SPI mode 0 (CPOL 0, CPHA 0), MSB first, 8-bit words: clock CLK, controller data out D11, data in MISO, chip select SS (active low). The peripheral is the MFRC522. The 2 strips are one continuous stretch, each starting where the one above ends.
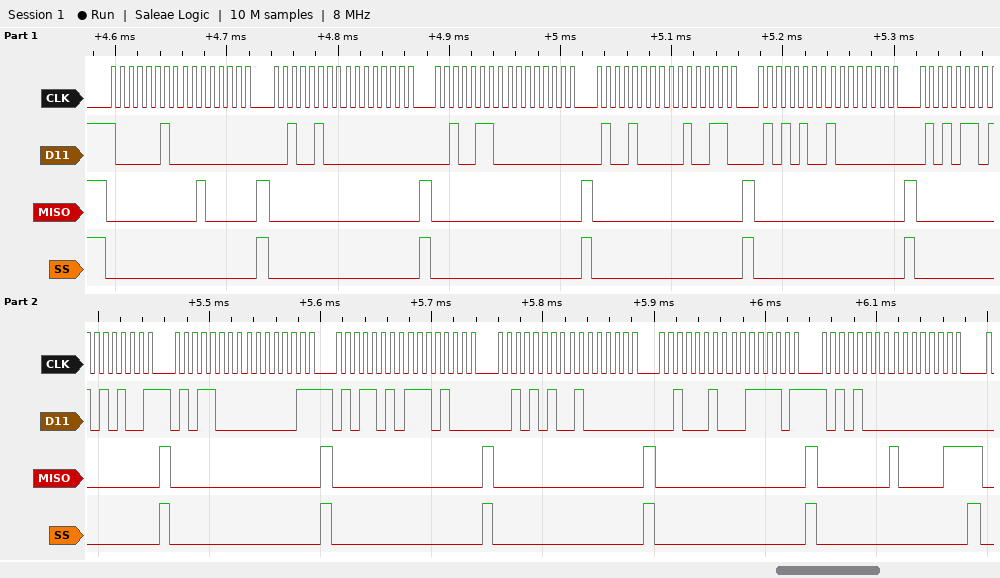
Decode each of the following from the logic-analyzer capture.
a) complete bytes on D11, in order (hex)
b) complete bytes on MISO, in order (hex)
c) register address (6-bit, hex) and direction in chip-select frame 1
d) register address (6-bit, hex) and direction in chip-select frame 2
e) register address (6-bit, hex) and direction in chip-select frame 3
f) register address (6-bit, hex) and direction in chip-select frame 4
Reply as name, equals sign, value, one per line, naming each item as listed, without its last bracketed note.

complete bytes on D11, in order = 82 00 24 00 26 00 48 26 54 80 56 A9 58 03 5A E8 2A 40 22 3D A8 00
complete bytes on MISO, in order = 00 20 00 00 00 00 00 00 00 00 00 00 00 00 00 00 00 00 00 00 00 83
register address (6-bit, hex) and direction in chip-select frame 1 = 0x01 read
register address (6-bit, hex) and direction in chip-select frame 2 = 0x12 write
register address (6-bit, hex) and direction in chip-select frame 3 = 0x13 write
register address (6-bit, hex) and direction in chip-select frame 4 = 0x24 write
